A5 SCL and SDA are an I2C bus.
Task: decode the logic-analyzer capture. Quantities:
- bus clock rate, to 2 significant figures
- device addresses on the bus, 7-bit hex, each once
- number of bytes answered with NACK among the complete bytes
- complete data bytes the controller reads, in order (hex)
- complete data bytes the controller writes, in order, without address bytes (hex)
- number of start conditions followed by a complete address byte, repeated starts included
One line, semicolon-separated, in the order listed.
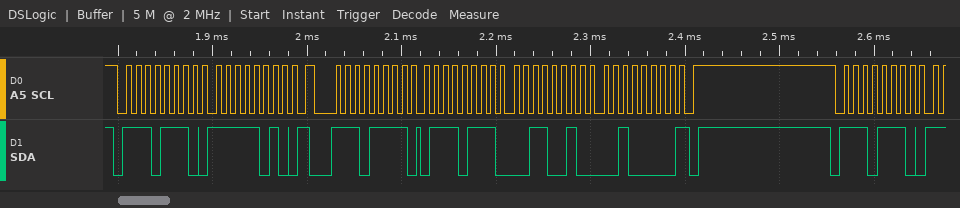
100 kHz; 0x77; 1; 77 32 20; FA; 3
